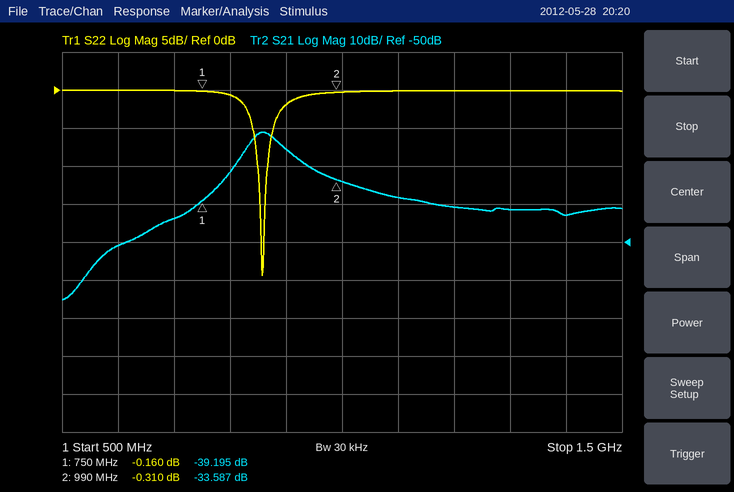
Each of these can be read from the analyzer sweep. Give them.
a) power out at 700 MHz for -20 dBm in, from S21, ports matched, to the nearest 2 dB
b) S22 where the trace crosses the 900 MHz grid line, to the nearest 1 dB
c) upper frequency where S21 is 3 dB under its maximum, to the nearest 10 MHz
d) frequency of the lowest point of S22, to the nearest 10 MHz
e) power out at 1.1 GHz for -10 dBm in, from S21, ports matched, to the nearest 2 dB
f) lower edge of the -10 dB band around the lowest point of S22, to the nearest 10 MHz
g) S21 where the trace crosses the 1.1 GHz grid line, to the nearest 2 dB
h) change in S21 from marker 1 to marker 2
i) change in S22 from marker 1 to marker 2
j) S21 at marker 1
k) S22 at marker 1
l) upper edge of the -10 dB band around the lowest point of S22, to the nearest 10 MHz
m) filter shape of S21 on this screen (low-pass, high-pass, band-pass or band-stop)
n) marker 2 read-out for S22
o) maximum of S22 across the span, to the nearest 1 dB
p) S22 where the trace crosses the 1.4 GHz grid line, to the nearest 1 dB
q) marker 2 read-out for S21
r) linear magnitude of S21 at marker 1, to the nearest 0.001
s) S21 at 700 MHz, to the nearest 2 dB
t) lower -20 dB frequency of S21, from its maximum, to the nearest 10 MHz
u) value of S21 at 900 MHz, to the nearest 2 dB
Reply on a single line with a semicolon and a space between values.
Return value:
-64 dBm; -2 dB; 890 MHz; 860 MHz; -48 dBm; 850 MHz; -38 dB; 5.608 dB; -0.150 dB; -39.195 dB; -0.160 dB; 870 MHz; band-pass; -0.310 dB; 0 dB; 0 dB; -33.587 dB; 0.011; -44 dB; 730 MHz; -26 dB
